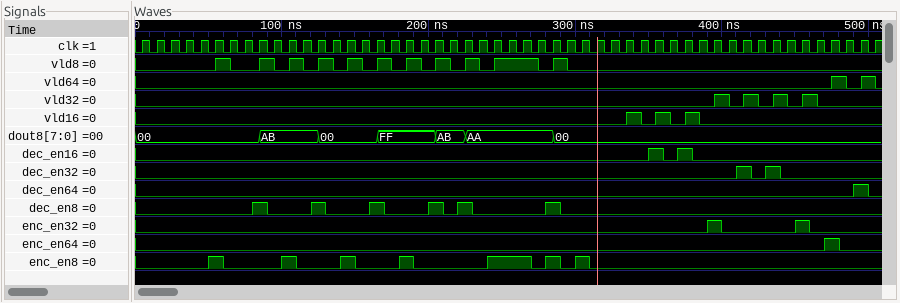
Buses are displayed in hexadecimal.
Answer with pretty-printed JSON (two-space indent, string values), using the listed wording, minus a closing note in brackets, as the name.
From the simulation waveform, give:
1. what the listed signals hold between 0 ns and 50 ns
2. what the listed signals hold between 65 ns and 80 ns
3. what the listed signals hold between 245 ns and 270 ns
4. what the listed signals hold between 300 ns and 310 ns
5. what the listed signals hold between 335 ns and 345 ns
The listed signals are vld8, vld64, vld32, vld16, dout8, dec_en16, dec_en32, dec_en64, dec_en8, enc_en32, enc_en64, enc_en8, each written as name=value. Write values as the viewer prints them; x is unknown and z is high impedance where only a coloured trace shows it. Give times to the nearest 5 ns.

{
  "what the listed signals hold between 0 ns and 50 ns": "vld8=0, vld64=0, vld32=0, vld16=0, dout8=00, dec_en16=0, dec_en32=0, dec_en64=0, dec_en8=0, enc_en32=0, enc_en64=0, enc_en8=0",
  "what the listed signals hold between 65 ns and 80 ns": "vld8=0, vld64=0, vld32=0, vld16=0, dout8=00, dec_en16=0, dec_en32=0, dec_en64=0, dec_en8=0, enc_en32=0, enc_en64=0, enc_en8=0",
  "what the listed signals hold between 245 ns and 270 ns": "vld8=1, vld64=0, vld32=0, vld16=0, dout8=AA, dec_en16=0, dec_en32=0, dec_en64=0, dec_en8=0, enc_en32=0, enc_en64=0, enc_en8=1",
  "what the listed signals hold between 300 ns and 310 ns": "vld8=0, vld64=0, vld32=0, vld16=0, dout8=00, dec_en16=0, dec_en32=0, dec_en64=0, dec_en8=0, enc_en32=0, enc_en64=0, enc_en8=1",
  "what the listed signals hold between 335 ns and 345 ns": "vld8=0, vld64=0, vld32=0, vld16=1, dout8=00, dec_en16=0, dec_en32=0, dec_en64=0, dec_en8=0, enc_en32=0, enc_en64=0, enc_en8=0"
}
